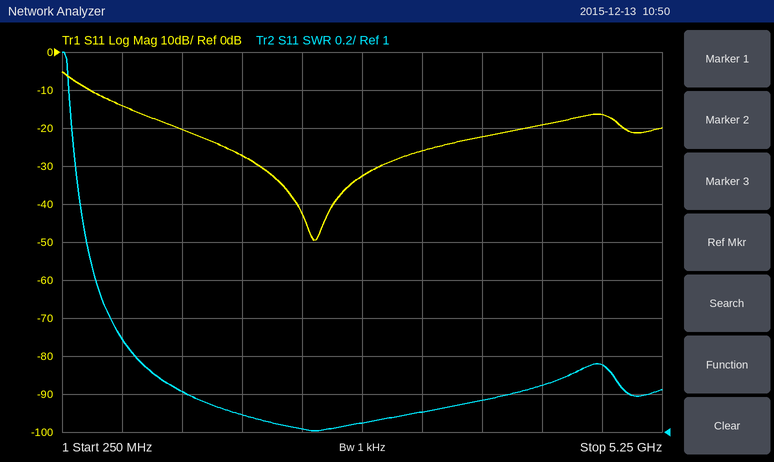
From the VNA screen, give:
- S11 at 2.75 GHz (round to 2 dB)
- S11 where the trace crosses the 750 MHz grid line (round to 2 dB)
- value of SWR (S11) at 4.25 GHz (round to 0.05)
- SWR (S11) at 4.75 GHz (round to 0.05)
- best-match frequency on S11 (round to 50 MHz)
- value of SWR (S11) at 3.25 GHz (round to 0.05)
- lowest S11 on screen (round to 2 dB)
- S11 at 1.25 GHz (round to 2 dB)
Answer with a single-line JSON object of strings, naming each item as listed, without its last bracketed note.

{"S11 at 2.75 GHz": "-32 dB", "S11 where the trace crosses the 750 MHz grid line": "-14 dB", "value of SWR (S11) at 4.25 GHz": "1.25", "SWR (S11) at 4.75 GHz": "1.35", "best-match frequency on S11": "2.35 GHz", "value of SWR (S11) at 3.25 GHz": "1.10", "lowest S11 on screen": "-50 dB", "S11 at 1.25 GHz": "-20 dB"}
